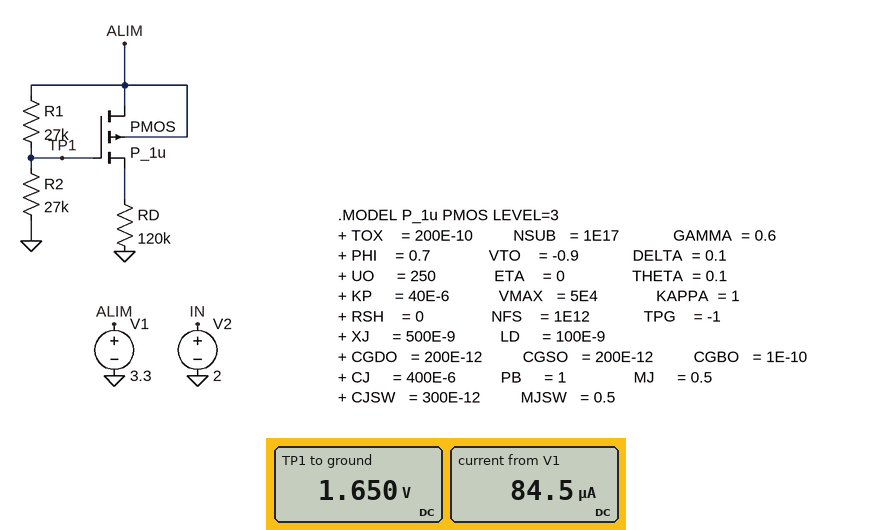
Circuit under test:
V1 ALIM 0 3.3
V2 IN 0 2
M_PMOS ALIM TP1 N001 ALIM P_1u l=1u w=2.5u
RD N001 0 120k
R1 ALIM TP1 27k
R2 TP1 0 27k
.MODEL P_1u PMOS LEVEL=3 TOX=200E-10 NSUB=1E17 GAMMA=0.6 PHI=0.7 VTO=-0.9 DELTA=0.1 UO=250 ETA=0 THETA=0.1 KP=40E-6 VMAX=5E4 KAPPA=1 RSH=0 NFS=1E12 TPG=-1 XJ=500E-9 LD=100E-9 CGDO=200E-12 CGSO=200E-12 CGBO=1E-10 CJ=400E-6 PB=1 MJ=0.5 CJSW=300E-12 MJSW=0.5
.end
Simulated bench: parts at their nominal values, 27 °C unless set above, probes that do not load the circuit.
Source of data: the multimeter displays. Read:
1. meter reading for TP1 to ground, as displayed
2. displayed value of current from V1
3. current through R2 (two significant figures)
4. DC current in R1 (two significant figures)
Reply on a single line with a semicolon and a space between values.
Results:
1.650 V; 84.5 µA; 61 µA; 61 µA
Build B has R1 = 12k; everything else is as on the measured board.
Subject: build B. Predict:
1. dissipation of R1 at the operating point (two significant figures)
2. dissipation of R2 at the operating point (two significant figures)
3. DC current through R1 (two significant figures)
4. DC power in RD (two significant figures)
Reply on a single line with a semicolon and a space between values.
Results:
86 µW; 190 µW; 85 µA; 370 nW
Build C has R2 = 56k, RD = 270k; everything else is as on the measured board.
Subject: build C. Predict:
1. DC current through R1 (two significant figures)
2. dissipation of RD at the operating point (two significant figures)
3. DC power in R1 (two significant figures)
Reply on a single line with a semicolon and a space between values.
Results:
40 µA; 2.4 µW; 43 µW
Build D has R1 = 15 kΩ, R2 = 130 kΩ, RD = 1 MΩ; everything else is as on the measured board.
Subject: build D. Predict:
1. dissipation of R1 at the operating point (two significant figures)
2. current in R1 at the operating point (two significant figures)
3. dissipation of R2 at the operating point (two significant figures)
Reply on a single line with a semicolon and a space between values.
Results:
7.8 µW; 23 µA; 67 µW
